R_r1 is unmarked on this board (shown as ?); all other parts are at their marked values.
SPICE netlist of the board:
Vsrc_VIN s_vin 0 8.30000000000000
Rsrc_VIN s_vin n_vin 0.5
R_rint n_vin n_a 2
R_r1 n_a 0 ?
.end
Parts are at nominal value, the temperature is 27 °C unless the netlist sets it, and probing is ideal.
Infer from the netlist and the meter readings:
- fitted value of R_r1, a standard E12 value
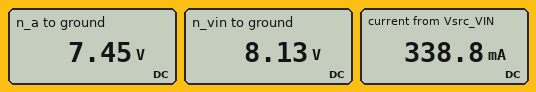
22 Ω
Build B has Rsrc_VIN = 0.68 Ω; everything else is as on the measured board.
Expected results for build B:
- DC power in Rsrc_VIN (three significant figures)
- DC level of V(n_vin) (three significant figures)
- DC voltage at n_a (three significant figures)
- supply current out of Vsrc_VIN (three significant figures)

76.9 mW
8.07 V
7.40 V
336 mA
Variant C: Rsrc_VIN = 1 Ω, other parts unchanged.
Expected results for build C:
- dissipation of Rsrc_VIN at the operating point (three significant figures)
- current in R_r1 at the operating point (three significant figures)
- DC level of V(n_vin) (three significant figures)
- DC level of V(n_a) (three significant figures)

110 mW
332 mA
7.97 V
7.30 V
